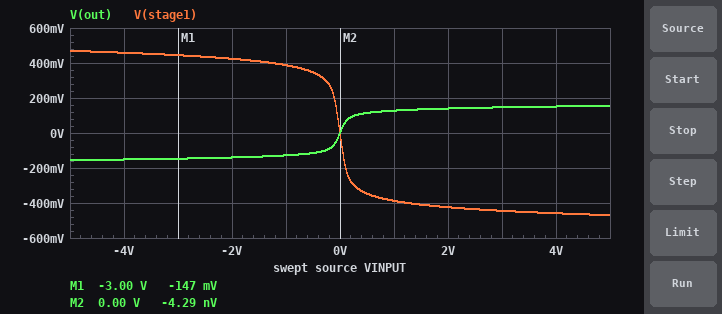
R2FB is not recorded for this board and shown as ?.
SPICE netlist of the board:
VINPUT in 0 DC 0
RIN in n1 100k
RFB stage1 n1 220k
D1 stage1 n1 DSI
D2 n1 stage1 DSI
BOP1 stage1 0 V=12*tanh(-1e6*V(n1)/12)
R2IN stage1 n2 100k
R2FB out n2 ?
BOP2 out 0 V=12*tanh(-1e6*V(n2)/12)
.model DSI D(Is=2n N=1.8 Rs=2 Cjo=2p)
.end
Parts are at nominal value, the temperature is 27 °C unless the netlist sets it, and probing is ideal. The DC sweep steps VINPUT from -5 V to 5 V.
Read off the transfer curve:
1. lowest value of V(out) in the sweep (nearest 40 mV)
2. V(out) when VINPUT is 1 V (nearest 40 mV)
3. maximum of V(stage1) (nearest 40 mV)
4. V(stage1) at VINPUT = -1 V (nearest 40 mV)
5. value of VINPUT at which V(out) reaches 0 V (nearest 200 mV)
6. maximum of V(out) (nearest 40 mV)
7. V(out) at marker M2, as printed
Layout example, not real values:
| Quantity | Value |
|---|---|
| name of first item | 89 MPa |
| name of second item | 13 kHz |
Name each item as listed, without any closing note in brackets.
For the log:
| Quantity | Value |
|---|---|
| lowest value of V(out) in the sweep | -160 mV |
| V(out) when VINPUT is 1 V | 120 mV |
| maximum of V(stage1) | 480 mV |
| V(stage1) at VINPUT = -1 V | 400 mV |
| value of VINPUT at which V(out) reaches 0 V | 0 V |
| maximum of V(out) | 160 mV |
| V(out) at marker M2, as printed | -4.29 nV |
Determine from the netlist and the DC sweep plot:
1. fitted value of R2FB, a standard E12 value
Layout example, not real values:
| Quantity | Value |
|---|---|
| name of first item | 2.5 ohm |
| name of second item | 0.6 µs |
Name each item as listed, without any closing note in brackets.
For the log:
| Quantity | Value |
|---|---|
| fitted value of R2FB, a standard E12 value | 33 kΩ |
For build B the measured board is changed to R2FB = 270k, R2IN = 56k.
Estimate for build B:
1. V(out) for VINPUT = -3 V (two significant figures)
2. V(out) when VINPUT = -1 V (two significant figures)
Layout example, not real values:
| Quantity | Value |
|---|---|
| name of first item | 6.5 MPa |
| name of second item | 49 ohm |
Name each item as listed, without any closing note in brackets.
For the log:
| Quantity | Value |
|---|---|
| V(out) for VINPUT = -3 V | -2.1 V |
| V(out) when VINPUT = -1 V | -1.9 V |
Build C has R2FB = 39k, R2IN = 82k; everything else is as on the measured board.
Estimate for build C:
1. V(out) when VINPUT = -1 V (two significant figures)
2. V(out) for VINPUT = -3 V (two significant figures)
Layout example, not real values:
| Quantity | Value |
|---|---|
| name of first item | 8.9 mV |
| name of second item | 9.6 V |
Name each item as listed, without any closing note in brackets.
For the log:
| Quantity | Value |
|---|---|
| V(out) when VINPUT = -1 V | -180 mV |
| V(out) for VINPUT = -3 V | -210 mV |
